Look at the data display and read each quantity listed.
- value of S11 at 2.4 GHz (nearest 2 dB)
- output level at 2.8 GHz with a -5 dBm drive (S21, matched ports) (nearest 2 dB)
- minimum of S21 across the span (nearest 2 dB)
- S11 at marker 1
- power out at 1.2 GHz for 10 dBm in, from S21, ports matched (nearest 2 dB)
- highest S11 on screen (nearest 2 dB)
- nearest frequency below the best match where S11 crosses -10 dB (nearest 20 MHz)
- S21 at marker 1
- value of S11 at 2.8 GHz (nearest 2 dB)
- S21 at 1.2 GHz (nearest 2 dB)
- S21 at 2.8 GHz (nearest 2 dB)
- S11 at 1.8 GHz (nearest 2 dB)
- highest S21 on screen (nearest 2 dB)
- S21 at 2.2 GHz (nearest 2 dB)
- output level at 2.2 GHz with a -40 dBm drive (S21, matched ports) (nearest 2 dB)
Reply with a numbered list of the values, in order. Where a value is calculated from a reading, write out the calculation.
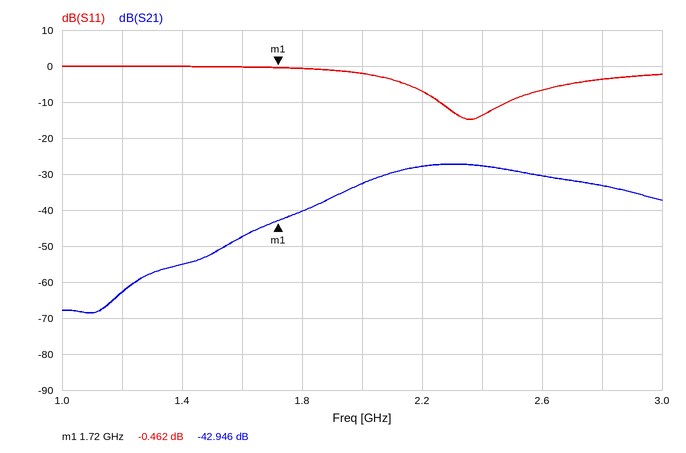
1. -14 dB
2. -5 dBm + (-34 dB) = -38 dBm
3. -68 dB
4. -0.462 dB
5. 10 dBm + (-62 dB) = -52 dBm
6. 0 dB
7. 2.26 GHz
8. -42.946 dB
9. -4 dB
10. -62 dB
11. -34 dB
12. 0 dB
13. -28 dB
14. -28 dB
15. -40 dBm + (-28 dB) = -68 dBm
